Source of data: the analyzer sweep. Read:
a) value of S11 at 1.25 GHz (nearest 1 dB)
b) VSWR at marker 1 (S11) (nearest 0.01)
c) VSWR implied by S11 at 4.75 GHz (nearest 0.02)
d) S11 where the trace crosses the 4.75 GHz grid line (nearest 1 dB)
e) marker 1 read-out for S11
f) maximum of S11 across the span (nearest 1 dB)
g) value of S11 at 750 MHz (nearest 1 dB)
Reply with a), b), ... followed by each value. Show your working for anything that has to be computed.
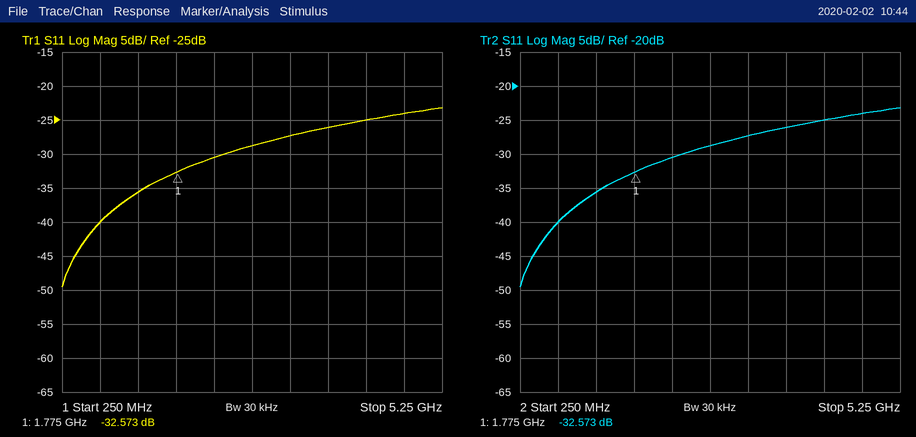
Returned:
a) -36 dB
b) (1 + 0.0235)/(1 − 0.0235) ≈ 1.05
c) |Γ| = 10^(-24/20) = 0.0631; VSWR = (1 + 0.0631)/(1 − 0.0631) ≈ 1.13, so 1.14 to the nearest 0.02
d) -24 dB
e) -32.573 dB
f) -23 dB
g) -40 dB
